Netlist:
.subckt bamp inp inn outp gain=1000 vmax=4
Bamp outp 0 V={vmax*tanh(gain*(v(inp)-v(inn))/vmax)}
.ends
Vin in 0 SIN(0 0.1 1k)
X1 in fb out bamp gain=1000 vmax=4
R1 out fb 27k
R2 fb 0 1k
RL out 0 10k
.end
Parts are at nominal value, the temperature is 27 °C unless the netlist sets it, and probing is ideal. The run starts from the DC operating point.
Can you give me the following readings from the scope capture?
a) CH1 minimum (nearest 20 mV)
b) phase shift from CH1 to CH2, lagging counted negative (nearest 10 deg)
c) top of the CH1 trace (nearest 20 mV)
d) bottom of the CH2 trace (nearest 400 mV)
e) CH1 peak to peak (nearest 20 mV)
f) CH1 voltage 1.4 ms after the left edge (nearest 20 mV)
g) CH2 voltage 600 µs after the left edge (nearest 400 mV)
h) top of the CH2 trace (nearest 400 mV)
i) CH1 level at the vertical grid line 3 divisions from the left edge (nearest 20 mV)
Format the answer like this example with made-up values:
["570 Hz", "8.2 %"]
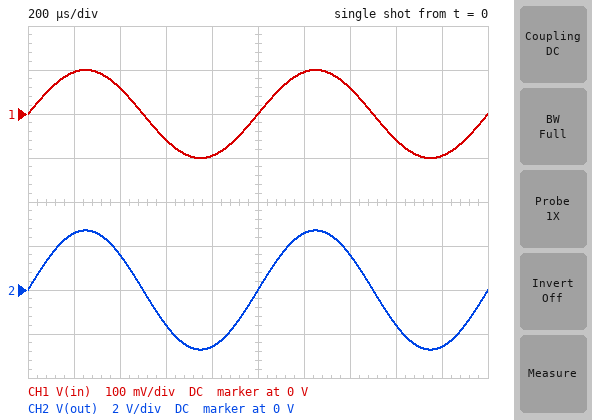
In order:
["-100 mV", "0 deg", "100 mV", "-2.8 V", "200 mV", "60 mV", "-1.6 V", "2.8 V", "-60 mV"]
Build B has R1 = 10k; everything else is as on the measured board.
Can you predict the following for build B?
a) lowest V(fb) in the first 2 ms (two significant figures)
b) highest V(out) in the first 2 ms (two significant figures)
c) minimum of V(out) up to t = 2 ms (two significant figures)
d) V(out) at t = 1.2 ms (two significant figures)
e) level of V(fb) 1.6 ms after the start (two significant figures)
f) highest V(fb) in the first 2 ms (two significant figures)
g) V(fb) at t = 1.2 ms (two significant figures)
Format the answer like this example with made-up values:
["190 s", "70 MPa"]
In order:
["-99 mV", "1.1 V", "-1.1 V", "1.0 V", "-58 mV", "99 mV", "94 mV"]
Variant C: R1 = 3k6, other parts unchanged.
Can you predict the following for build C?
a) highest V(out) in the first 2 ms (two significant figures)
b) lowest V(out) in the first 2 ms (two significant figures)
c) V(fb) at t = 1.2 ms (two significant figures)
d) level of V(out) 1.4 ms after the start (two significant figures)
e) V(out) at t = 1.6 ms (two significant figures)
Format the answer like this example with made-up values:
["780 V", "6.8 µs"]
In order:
["460 mV", "-460 mV", "95 mV", "270 mV", "-270 mV"]
